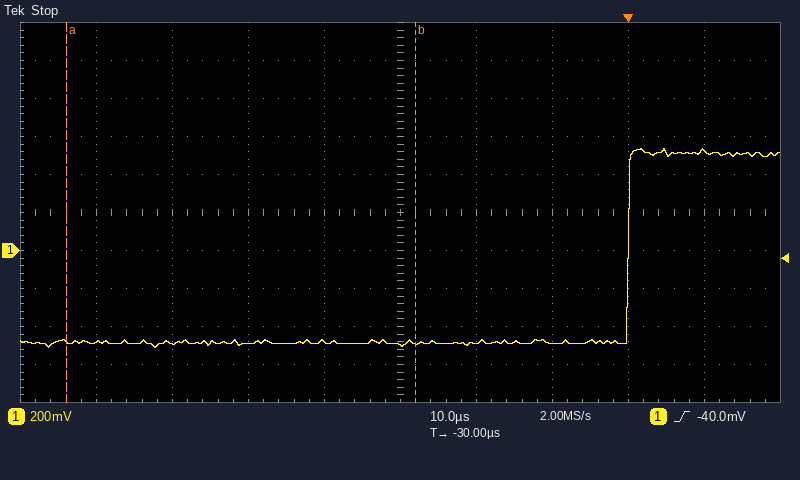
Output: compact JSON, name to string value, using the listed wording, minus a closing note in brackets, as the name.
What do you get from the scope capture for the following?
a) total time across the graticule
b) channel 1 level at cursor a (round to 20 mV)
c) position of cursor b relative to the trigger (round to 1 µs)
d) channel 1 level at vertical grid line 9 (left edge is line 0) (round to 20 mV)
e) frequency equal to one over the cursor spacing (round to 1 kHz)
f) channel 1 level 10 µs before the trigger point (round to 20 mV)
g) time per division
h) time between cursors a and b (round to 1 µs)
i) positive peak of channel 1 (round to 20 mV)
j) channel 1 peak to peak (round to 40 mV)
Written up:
{"total time across the graticule": "100 µs", "channel 1 level at cursor a": "-480 mV", "position of cursor b relative to the trigger": "-28 µs", "channel 1 level at vertical grid line 9 (left edge is line 0)": "520 mV", "frequency equal to one over the cursor spacing": "22 kHz", "channel 1 level 10 µs before the trigger point": "-480 mV", "time per division": "10 µs", "time between cursors a and b": "46 µs", "positive peak of channel 1": "540 mV", "channel 1 peak to peak": "1.04 V"}
